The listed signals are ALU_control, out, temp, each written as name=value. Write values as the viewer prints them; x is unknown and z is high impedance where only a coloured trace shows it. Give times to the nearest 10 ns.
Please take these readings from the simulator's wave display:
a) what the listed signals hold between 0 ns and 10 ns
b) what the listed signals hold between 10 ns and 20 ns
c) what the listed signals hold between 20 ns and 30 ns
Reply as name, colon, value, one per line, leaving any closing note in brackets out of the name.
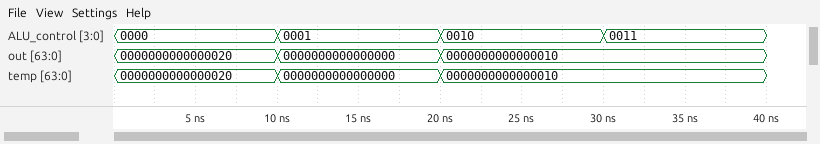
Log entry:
what the listed signals hold between 0 ns and 10 ns: ALU_control=0000, out=0000000000000020, temp=0000000000000020
what the listed signals hold between 10 ns and 20 ns: ALU_control=0001, out=0000000000000000, temp=0000000000000000
what the listed signals hold between 20 ns and 30 ns: ALU_control=0010, out=0000000000000010, temp=0000000000000010
